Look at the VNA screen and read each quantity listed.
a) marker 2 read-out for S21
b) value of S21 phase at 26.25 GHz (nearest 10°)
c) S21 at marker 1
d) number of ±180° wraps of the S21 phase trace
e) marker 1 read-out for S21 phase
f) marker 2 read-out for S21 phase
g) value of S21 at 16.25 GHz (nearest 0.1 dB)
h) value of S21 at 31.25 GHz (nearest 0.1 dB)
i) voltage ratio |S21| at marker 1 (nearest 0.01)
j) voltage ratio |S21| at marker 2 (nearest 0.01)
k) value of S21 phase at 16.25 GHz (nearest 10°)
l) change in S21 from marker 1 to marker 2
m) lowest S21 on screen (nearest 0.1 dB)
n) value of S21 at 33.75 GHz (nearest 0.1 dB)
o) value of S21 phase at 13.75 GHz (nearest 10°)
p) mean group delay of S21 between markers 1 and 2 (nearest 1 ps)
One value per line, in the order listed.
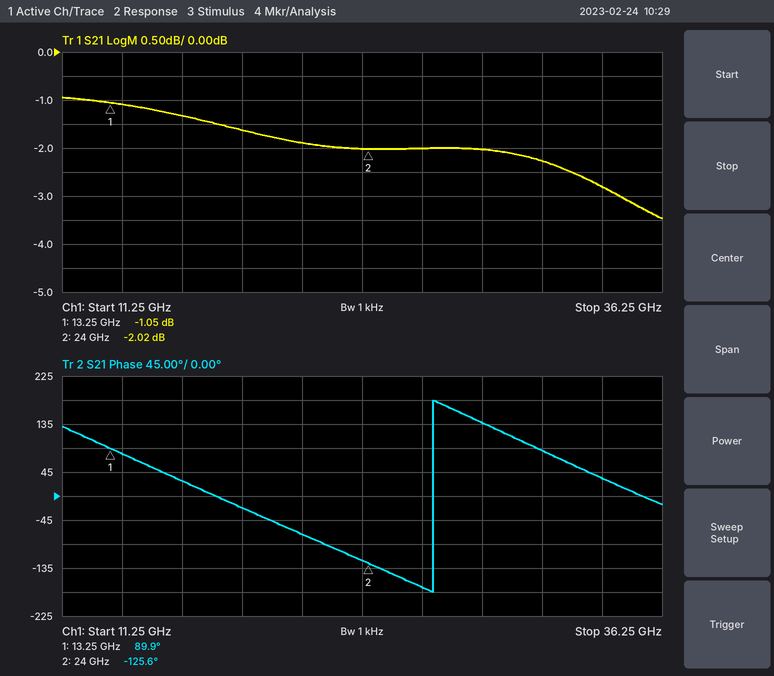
-2.02 dB
-170°
-1.05 dB
1
89.9°
-125.6°
-1.3 dB
-2.3 dB
0.89
0.79
30°
-0.97 dB
-3.5 dB
-2.8 dB
80°
56 ps
